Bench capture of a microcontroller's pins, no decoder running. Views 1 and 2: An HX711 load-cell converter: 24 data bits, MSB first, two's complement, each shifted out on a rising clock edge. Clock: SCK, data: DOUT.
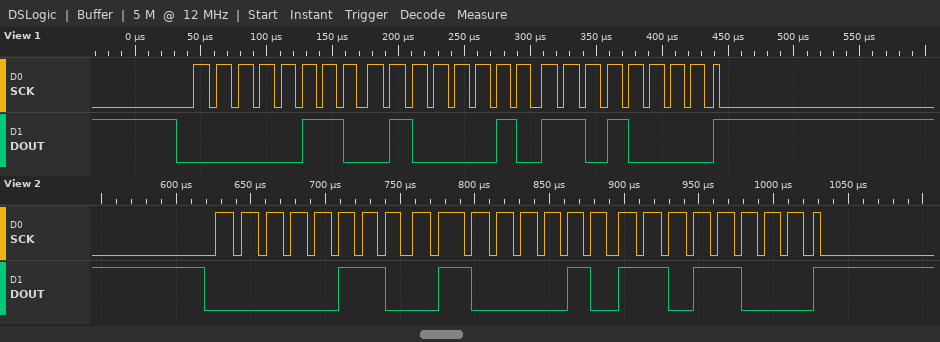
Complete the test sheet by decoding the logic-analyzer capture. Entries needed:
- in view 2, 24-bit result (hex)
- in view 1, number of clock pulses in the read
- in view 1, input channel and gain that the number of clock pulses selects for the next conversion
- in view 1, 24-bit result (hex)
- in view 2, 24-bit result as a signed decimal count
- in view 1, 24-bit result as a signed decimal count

0x0642D8
25
channel A, gain 128
0x0642D0
410328
410320
